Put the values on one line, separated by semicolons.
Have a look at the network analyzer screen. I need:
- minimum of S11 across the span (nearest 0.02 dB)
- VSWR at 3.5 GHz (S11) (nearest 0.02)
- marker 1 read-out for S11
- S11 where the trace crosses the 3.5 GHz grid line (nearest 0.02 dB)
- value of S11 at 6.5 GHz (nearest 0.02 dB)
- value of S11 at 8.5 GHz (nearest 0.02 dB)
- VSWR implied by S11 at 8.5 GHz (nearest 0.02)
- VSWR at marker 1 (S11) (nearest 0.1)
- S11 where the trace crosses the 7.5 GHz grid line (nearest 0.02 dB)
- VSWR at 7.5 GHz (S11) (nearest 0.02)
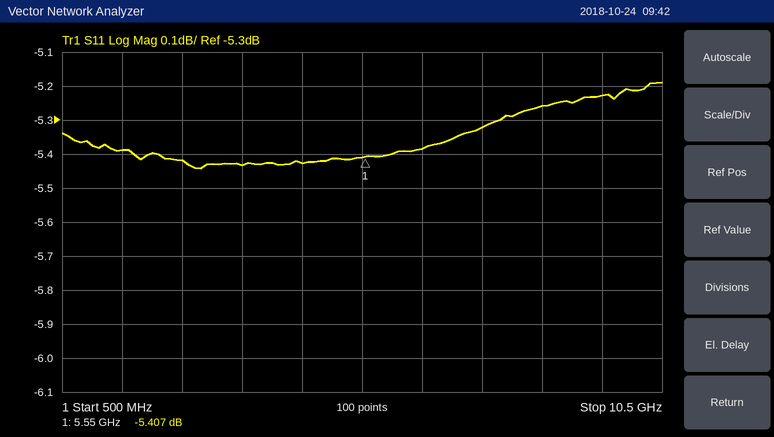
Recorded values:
-5.44 dB; 3.30; -5.407 dB; -5.44 dB; -5.38 dB; -5.26 dB; 3.40; 3.3; -5.32 dB; 3.36
